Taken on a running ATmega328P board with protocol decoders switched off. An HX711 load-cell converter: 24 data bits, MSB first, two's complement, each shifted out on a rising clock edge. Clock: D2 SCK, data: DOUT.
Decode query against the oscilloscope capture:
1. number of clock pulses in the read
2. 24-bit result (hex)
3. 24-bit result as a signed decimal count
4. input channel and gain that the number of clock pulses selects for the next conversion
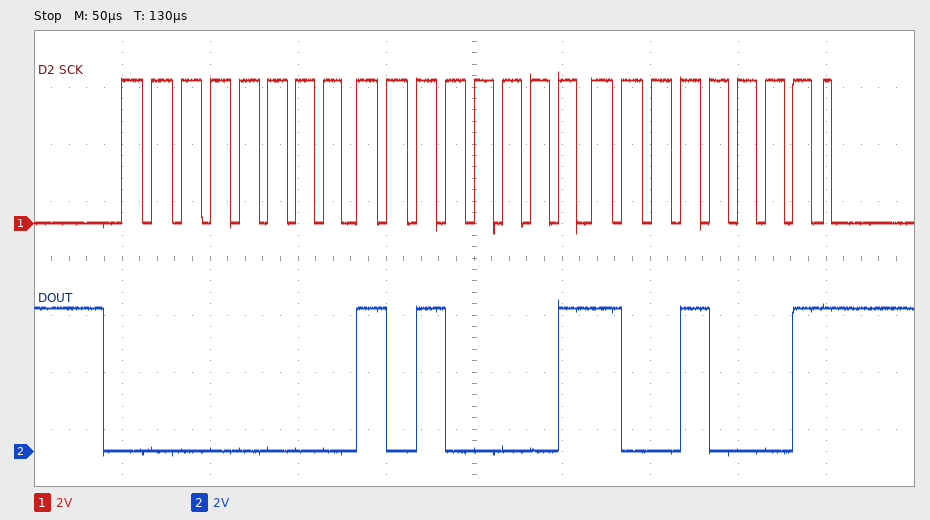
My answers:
25
0x00A191
41361
channel A, gain 128
